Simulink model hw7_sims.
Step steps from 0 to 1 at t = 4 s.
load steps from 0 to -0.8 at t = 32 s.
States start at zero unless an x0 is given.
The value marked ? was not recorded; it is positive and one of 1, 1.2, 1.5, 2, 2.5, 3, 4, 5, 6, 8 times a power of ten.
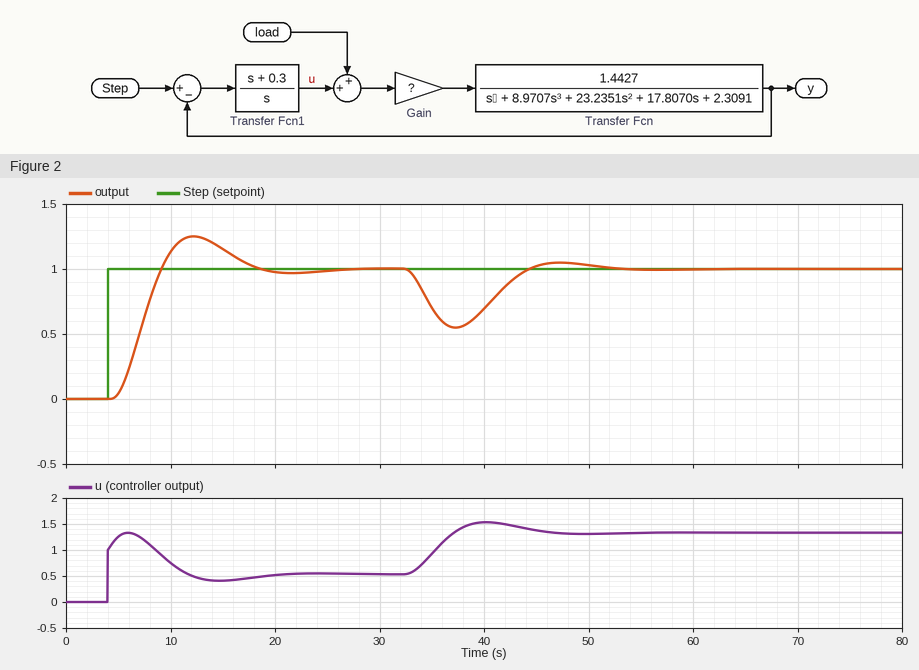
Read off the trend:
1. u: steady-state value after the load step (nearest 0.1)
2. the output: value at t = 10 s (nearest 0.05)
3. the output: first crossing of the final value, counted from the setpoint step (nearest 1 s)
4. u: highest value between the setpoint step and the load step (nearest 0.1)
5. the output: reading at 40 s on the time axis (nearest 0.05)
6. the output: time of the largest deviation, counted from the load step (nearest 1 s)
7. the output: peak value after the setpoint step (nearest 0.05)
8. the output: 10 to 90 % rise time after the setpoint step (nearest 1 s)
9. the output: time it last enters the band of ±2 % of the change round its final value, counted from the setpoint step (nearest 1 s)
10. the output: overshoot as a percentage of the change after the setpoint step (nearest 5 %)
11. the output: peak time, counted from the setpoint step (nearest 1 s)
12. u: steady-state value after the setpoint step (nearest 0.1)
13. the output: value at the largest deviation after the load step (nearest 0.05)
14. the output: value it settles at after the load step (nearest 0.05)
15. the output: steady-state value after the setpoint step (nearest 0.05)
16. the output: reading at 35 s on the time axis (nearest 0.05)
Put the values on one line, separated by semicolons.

1.3; 1.15; 5 s; 1.3; 0.70; 5 s; 1.25; 3 s; 20 s; 25 %; 8 s; 0.5; 0.55; 1.00; 1.00; 0.70
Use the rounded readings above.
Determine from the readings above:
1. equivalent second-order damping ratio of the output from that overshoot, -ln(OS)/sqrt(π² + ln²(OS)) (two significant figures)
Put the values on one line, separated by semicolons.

0.40
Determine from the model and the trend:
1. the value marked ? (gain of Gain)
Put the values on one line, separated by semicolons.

3
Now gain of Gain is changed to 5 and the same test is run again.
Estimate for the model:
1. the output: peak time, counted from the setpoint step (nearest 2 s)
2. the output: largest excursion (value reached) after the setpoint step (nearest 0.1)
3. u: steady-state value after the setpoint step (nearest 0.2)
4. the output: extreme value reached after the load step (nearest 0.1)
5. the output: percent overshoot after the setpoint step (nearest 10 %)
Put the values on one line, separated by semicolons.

6 s; 1.4; 0.4; 0.4; 40 %
